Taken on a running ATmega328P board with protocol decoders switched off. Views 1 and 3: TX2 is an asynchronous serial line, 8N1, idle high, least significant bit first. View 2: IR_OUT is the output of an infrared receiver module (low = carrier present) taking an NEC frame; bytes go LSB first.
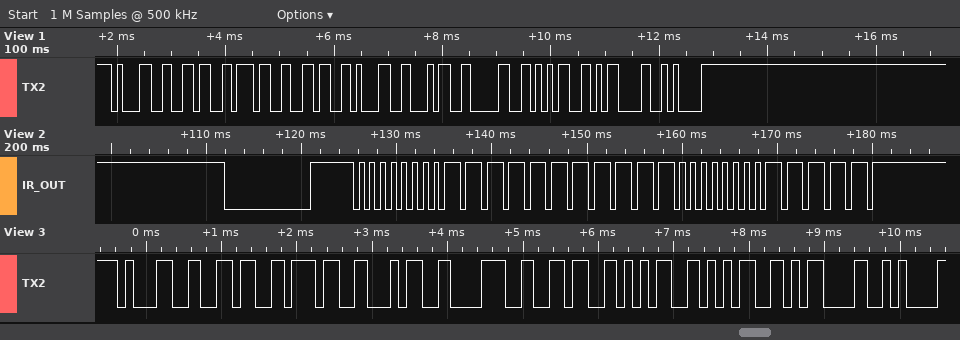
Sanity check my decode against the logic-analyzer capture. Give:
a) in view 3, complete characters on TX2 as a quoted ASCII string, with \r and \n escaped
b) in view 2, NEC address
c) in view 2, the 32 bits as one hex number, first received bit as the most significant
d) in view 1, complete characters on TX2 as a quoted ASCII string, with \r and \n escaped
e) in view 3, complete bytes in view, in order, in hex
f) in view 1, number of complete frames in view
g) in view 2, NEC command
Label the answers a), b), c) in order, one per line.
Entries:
a) "16748655\r\n"
b) 0x00
c) 0x00FFE01F
d) "16761405\r\n"
e) 0x31 0x36 0x37 0x34 0x38 0x36 0x35 0x35 0x0D 0x0A
f) 10
g) 0x07
